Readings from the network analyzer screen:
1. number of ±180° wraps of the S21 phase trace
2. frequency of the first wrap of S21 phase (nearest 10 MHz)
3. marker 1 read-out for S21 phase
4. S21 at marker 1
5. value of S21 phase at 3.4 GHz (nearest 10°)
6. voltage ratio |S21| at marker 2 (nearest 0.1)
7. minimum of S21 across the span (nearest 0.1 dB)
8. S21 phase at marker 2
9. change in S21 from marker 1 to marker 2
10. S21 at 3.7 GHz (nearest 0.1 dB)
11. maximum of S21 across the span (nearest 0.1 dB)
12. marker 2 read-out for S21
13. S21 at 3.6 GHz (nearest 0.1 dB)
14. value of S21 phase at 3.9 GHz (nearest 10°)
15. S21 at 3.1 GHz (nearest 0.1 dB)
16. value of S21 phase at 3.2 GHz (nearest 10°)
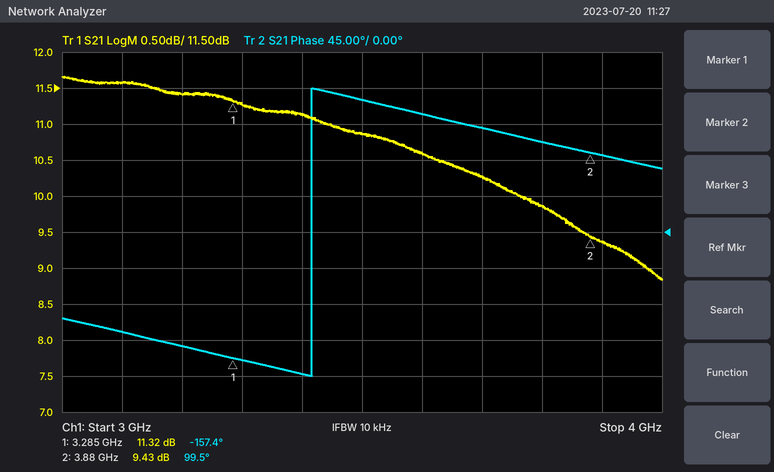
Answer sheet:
1
3.42 GHz
-157.4°
11.32 dB
-180°
3.0
8.8 dB
99.5°
-1.89 dB
10.3 dB
11.7 dB
9.43 dB
10.6 dB
100°
11.6 dB
-140°
